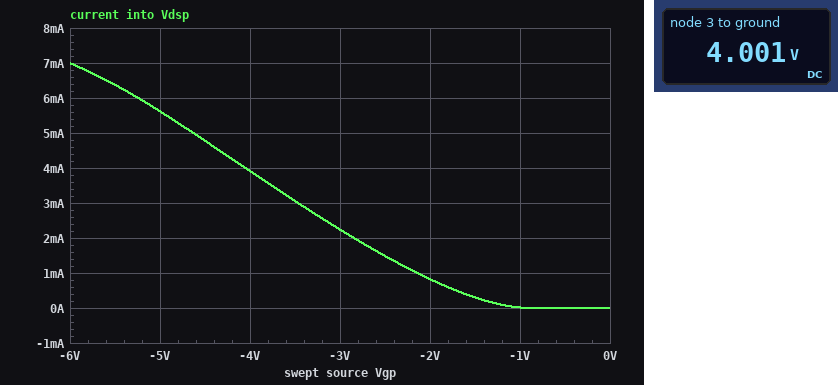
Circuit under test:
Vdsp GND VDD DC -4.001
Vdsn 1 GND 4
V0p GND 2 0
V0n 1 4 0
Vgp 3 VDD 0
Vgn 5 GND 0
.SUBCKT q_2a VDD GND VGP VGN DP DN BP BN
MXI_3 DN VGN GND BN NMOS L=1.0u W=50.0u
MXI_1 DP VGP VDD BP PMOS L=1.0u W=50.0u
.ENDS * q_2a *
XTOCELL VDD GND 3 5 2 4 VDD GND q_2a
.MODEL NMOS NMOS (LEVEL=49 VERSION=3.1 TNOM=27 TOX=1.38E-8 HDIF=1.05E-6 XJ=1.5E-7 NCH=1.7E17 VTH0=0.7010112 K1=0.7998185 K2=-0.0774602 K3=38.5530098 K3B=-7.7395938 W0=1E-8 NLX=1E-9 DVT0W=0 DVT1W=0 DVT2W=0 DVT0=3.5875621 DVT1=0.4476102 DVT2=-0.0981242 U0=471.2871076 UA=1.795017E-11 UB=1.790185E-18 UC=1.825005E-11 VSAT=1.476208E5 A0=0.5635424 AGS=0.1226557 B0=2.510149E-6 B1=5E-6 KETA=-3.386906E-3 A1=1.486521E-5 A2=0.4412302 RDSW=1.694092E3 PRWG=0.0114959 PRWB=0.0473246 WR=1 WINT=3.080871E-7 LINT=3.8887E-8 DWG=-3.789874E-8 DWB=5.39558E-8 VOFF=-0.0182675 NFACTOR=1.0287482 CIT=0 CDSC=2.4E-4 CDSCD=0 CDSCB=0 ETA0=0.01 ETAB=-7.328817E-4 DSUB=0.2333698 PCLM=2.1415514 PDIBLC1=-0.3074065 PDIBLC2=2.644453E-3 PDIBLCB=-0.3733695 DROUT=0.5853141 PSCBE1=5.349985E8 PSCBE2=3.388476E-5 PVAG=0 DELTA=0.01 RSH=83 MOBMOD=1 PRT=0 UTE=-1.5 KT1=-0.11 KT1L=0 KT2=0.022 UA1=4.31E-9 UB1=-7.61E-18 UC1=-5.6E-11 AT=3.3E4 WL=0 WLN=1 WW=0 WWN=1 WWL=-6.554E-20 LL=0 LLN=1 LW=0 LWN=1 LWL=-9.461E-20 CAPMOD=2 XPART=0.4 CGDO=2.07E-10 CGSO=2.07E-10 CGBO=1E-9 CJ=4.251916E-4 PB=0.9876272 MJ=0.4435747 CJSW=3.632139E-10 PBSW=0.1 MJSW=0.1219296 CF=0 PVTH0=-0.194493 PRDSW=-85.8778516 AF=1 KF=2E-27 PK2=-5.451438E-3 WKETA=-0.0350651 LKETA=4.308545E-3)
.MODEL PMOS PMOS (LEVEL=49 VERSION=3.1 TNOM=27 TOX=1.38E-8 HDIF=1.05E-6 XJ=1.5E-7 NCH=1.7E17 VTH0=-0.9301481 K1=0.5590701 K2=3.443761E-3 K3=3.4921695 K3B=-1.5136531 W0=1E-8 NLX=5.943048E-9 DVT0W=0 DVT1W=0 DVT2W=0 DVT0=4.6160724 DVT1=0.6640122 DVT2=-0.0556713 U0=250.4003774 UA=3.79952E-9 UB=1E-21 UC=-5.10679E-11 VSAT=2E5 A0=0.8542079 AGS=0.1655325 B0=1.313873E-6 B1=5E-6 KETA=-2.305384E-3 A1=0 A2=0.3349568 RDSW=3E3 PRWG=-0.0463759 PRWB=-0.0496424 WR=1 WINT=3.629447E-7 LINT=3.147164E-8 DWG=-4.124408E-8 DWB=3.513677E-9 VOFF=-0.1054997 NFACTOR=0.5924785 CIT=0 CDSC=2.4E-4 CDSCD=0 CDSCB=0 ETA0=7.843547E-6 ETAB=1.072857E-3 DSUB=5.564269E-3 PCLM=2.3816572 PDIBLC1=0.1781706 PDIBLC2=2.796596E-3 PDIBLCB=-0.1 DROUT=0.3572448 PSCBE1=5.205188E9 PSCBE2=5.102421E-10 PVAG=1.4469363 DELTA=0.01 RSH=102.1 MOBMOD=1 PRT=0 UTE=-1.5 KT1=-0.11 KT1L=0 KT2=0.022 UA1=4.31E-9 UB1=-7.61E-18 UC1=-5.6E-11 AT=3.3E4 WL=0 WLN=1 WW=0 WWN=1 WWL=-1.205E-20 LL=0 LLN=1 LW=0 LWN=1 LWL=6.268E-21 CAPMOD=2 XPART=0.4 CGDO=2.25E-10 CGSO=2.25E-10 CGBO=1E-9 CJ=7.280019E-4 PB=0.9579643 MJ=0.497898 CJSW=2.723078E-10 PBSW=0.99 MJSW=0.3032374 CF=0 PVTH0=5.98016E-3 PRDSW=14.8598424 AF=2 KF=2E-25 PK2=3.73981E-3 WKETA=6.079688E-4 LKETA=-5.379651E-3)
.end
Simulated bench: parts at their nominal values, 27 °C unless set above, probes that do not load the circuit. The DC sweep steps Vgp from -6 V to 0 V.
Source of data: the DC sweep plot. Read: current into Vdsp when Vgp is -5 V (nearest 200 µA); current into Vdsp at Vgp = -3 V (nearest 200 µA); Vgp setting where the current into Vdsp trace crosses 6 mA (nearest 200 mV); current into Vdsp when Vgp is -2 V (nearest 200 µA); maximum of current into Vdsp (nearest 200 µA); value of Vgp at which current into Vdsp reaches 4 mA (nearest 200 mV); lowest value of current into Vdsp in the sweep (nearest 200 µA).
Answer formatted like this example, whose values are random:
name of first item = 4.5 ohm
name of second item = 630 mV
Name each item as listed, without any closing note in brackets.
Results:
current into Vdsp when Vgp is -5 V = 5.6 mA
current into Vdsp at Vgp = -3 V = 2.2 mA
Vgp setting where the current into Vdsp trace crosses 6 mA = -5.2 V
current into Vdsp when Vgp is -2 V = 800 µA
maximum of current into Vdsp = 7.0 mA
value of Vgp at which current into Vdsp reaches 4 mA = -4.0 V
lowest value of current into Vdsp in the sweep = 0 A
